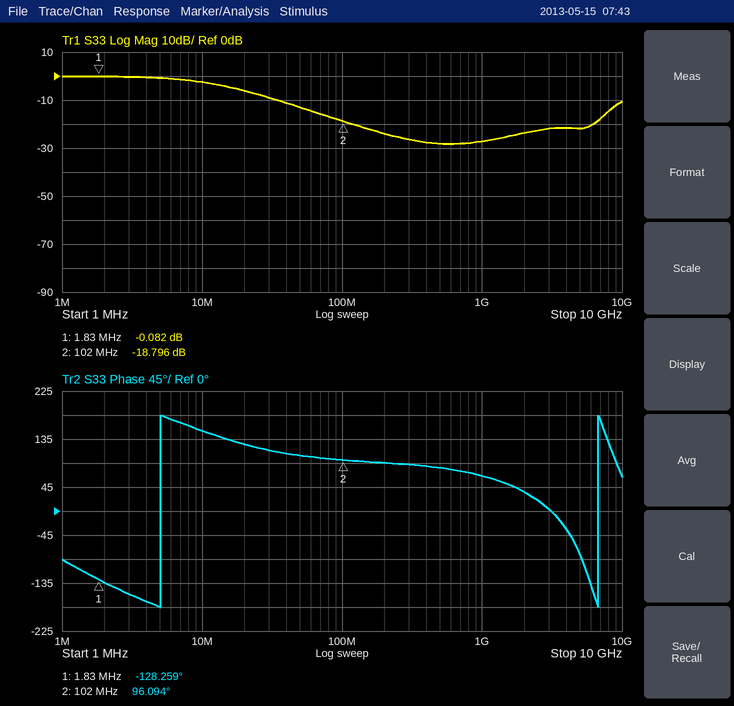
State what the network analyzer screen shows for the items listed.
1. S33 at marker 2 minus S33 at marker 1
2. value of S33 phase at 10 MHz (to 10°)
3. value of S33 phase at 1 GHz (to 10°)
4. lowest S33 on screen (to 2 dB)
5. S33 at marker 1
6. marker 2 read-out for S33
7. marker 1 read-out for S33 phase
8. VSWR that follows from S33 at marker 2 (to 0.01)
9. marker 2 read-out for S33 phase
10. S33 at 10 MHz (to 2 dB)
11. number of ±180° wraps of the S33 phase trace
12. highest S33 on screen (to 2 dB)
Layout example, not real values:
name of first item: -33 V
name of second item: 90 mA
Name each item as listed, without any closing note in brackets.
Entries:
S33 at marker 2 minus S33 at marker 1: -18.714 dB
value of S33 phase at 10 MHz: 150°
value of S33 phase at 1 GHz: 70°
lowest S33 on screen: -28 dB
S33 at marker 1: -0.082 dB
marker 2 read-out for S33: -18.796 dB
marker 1 read-out for S33 phase: -128.259°
VSWR that follows from S33 at marker 2: 1.26
marker 2 read-out for S33 phase: 96.094°
S33 at 10 MHz: -2 dB
number of ±180° wraps of the S33 phase trace: 2
highest S33 on screen: 0 dB
